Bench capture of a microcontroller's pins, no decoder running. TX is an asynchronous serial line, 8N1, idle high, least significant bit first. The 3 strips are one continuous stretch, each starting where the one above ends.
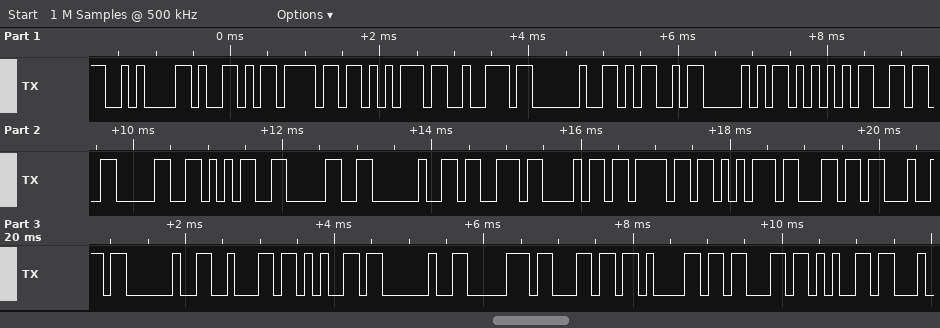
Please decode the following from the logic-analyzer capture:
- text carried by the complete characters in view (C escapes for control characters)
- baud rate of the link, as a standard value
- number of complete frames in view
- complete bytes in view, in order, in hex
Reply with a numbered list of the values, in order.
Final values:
1. "\nYour MPU6050 should be place"
2. 9600 baud
3. 29
4. 0x0A 0x59 0x6F 0x75 0x72 0x20 0x4D 0x50 0x55 0x36 0x30 0x35 0x30 0x20 0x73 0x68 0x6F 0x75 0x6C 0x64 0x20 0x62 0x65 0x20 0x70 0x6C 0x61 0x63 0x65
